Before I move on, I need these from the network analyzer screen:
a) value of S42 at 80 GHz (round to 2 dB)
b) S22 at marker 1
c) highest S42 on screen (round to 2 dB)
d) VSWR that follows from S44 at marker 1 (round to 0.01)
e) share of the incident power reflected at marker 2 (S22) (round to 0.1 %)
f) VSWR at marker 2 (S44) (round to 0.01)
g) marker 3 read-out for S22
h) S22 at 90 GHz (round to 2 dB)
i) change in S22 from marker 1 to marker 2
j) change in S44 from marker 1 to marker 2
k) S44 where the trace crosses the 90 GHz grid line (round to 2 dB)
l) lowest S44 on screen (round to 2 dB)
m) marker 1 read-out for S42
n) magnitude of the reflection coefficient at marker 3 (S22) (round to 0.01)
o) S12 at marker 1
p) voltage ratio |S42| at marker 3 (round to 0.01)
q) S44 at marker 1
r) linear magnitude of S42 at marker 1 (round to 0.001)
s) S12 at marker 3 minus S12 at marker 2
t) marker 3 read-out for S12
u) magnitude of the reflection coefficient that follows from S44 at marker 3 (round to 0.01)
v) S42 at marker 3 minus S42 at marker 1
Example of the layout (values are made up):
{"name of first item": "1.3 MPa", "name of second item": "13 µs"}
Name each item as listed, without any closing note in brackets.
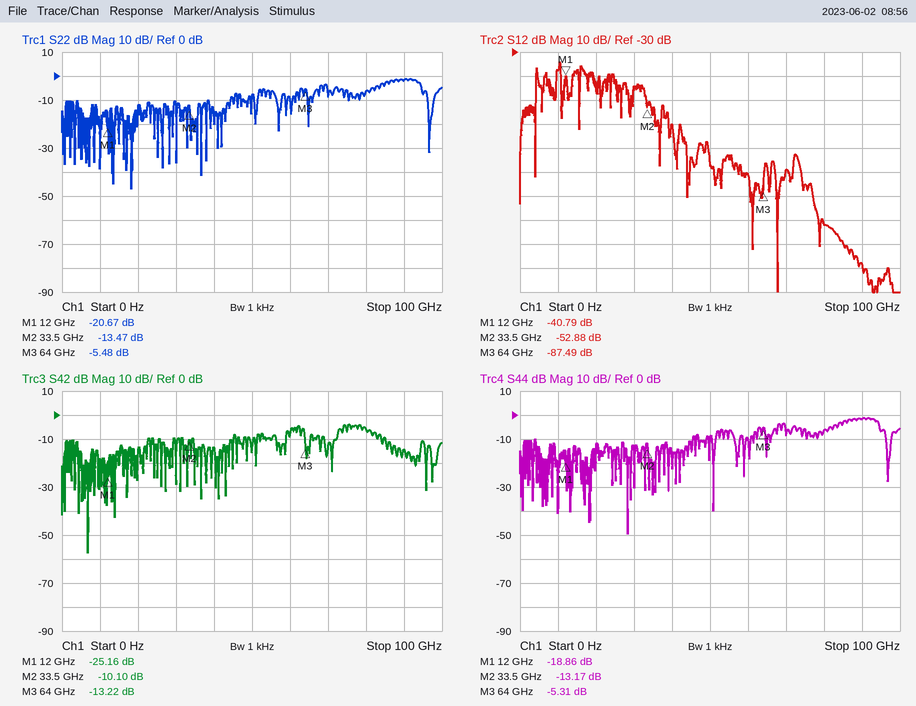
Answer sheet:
{"value of S42 at 80 GHz": "-6 dB", "S22 at marker 1": "-20.67 dB", "highest S42 on screen": "-4 dB", "VSWR that follows from S44 at marker 1": "1.26", "share of the incident power reflected at marker 2 (S22)": "4.5 %", "VSWR at marker 2 (S44)": "1.56", "marker 3 read-out for S22": "-5.48 dB", "S22 at 90 GHz": "-2 dB", "change in S22 from marker 1 to marker 2": "7.20 dB", "change in S44 from marker 1 to marker 2": "5.69 dB", "S44 where the trace crosses the 90 GHz grid line": "-2 dB", "lowest S44 on screen": "-50 dB", "marker 1 read-out for S42": "-25.16 dB", "magnitude of the reflection coefficient at marker 3 (S22)": "0.53", "S12 at marker 1": "-40.79 dB", "voltage ratio |S42| at marker 3": "0.22", "S44 at marker 1": "-18.86 dB", "linear magnitude of S42 at marker 1": "0.055", "S12 at marker 3 minus S12 at marker 2": "-34.61 dB", "marker 3 read-out for S12": "-87.49 dB", "magnitude of the reflection coefficient that follows from S44 at marker 3": "0.54", "S42 at marker 3 minus S42 at marker 1": "11.94 dB"}
